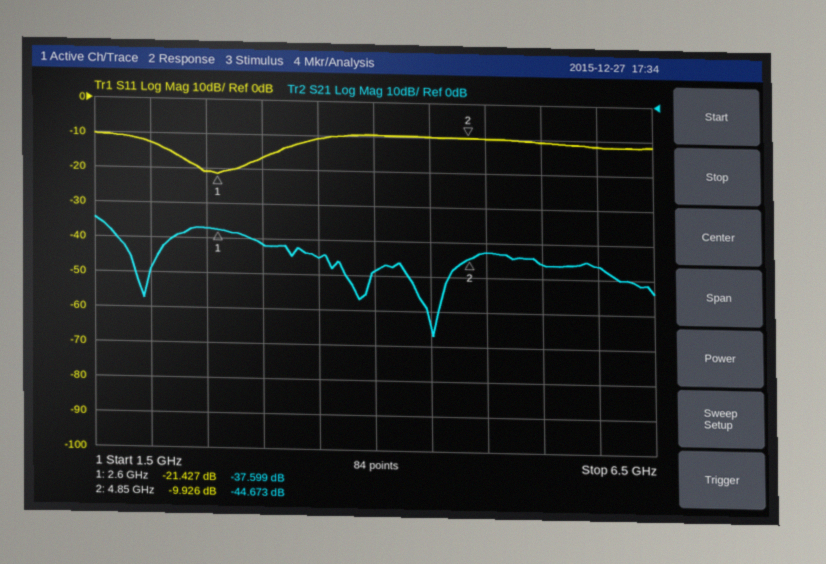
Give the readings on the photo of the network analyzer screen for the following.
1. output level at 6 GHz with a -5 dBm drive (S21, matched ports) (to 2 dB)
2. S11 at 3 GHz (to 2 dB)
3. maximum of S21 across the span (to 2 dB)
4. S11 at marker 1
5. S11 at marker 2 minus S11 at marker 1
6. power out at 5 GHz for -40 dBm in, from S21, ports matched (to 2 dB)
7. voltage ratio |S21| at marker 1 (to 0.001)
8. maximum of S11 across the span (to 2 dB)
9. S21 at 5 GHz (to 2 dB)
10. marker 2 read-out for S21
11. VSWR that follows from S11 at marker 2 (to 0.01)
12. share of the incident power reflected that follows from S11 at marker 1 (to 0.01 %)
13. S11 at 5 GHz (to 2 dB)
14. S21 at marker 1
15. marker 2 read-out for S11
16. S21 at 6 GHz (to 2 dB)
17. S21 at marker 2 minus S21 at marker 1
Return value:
-52 dBm
-16 dB
-34 dB
-21.427 dB
11.501 dB
-82 dBm
0.013
-10 dB
-42 dB
-44.673 dB
1.94
0.72 %
-10 dB
-37.599 dB
-9.926 dB
-46 dB
-7.074 dB
